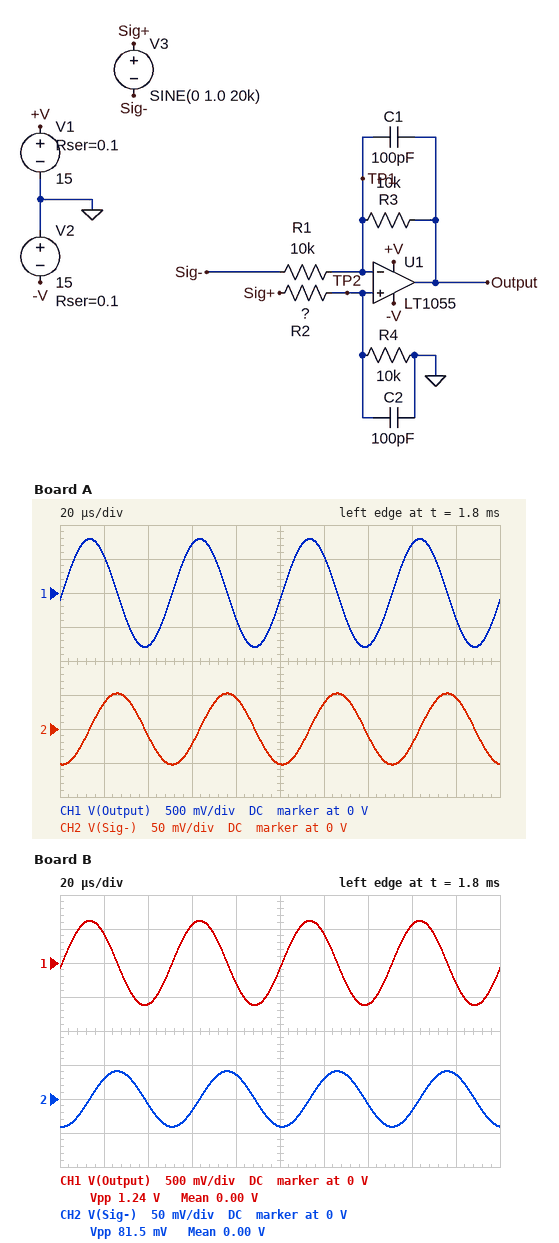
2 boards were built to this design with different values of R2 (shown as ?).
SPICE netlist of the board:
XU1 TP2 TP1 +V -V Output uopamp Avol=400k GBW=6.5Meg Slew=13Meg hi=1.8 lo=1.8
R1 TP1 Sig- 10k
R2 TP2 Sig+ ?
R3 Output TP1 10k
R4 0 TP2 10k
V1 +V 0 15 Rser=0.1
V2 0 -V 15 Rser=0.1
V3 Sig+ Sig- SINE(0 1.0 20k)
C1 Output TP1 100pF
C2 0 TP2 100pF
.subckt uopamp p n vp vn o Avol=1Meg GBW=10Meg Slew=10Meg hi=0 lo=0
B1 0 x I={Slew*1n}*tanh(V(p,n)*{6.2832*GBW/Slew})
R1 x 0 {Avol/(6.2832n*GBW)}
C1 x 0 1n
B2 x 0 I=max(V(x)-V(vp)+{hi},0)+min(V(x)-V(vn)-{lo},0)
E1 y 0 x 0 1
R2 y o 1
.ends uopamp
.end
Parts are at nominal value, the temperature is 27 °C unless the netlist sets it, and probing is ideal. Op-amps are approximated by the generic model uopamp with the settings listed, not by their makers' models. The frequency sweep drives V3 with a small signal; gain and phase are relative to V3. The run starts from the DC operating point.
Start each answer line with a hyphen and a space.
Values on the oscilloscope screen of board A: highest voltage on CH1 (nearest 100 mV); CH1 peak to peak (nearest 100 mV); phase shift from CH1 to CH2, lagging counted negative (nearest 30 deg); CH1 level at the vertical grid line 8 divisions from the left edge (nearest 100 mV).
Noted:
- 800 mV
- 1.6 V
- -90 deg
- 700 mV
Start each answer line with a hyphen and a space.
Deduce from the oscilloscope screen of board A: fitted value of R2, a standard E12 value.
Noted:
- 15 kΩ
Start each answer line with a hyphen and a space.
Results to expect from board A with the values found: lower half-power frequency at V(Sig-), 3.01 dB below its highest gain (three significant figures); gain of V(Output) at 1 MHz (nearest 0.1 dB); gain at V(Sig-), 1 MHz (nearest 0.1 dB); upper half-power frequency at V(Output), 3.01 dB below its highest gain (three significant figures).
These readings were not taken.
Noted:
- 154 kHz
- -18.3 dB
- -7.8 dB
- 156 kHz
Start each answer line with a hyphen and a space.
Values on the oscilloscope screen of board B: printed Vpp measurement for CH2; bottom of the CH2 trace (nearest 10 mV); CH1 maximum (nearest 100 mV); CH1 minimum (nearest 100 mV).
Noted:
- 81.5 mV
- -40 mV
- 600 mV
- -600 mV
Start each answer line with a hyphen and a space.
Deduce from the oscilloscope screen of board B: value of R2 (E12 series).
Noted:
- 22 kΩ
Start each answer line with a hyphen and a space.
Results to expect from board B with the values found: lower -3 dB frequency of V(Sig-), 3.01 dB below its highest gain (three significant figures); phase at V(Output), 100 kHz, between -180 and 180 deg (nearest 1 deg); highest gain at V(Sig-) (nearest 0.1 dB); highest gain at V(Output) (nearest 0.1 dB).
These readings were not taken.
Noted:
- 155 kHz
- -33 deg
- -9.9 dB
- -4.1 dB
